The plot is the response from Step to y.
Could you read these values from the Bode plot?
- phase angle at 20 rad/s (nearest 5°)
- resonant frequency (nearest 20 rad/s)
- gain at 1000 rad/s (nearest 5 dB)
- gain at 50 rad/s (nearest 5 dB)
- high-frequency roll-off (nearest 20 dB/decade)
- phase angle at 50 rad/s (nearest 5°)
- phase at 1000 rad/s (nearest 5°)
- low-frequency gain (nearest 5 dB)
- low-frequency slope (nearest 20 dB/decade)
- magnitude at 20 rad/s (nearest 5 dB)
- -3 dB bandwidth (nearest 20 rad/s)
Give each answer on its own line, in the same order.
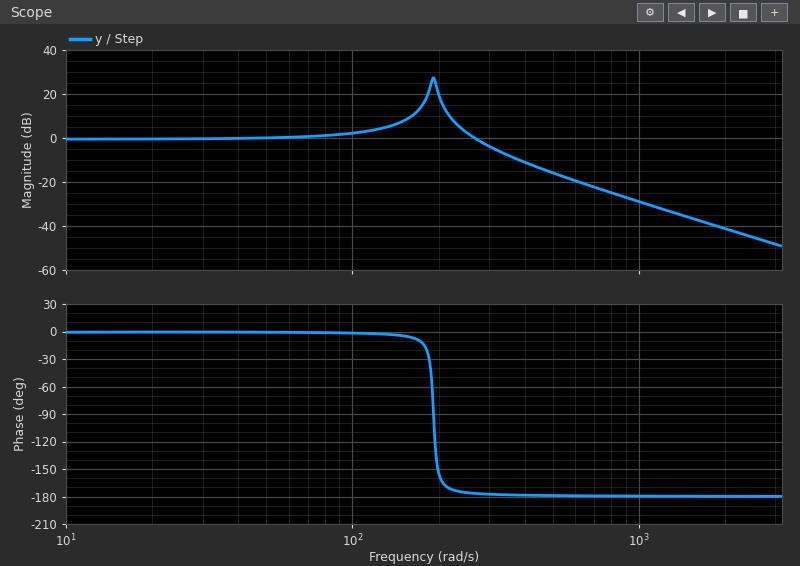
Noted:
0°
200 rad/s
-30 dB
0 dB
-40 dB/decade
0°
-180°
0 dB
0 dB/decade
0 dB
300 rad/s
